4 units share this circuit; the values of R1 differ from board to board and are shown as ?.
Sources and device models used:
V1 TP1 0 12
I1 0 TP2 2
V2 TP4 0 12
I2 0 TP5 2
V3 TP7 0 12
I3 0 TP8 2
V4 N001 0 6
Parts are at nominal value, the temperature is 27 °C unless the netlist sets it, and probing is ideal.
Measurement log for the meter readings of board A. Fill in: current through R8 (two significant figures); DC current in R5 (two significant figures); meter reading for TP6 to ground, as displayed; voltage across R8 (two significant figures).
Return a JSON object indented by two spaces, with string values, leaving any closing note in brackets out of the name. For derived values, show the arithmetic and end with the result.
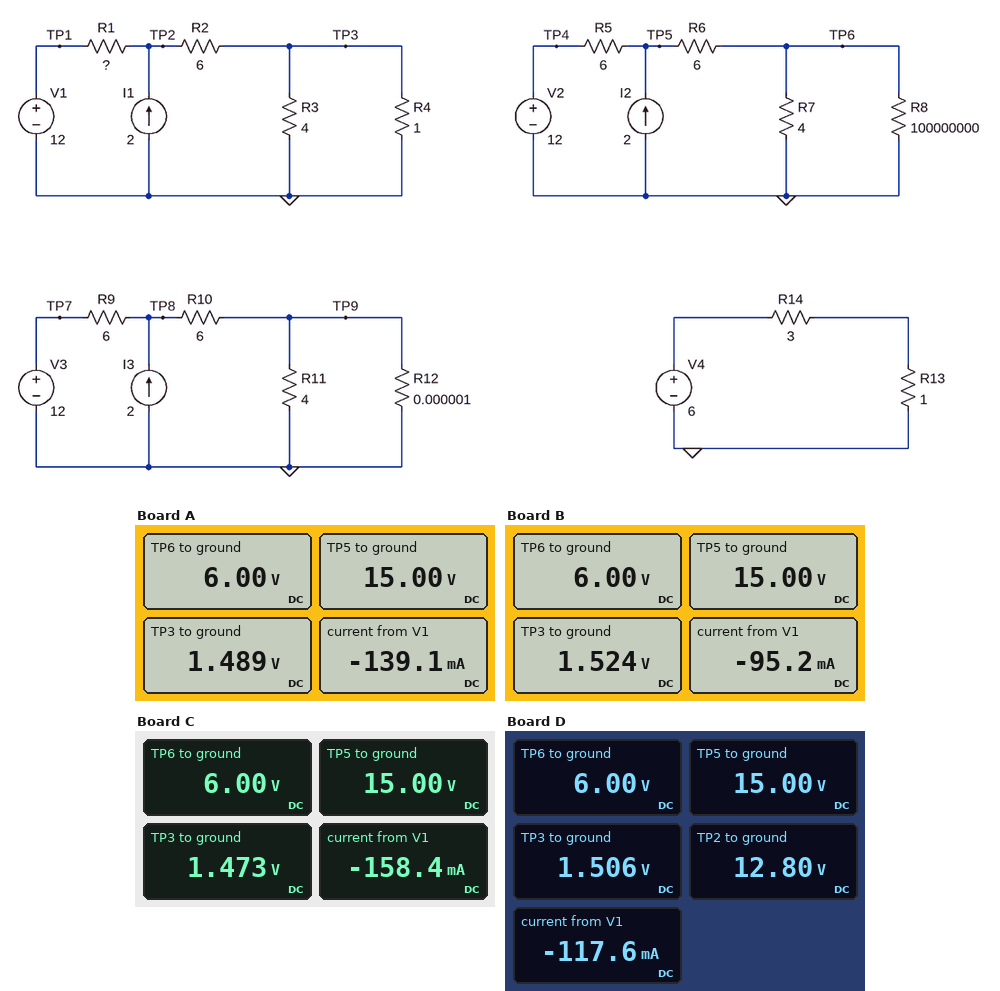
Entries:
{
  "current through R8": "(6 V) / 100 MΩ = 60 nA",
  "DC current in R5": "(15 V - 12 V) / 6 Ω = 500 mA",
  "meter reading for TP6 to ground, as displayed": "6.00 V",
  "voltage across R8": "6 V = 6.0 V"
}
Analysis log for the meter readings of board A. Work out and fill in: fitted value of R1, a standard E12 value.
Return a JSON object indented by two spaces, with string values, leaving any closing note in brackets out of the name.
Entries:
{
  "fitted value of R1, a standard E12 value": "4.7 Ω"
}
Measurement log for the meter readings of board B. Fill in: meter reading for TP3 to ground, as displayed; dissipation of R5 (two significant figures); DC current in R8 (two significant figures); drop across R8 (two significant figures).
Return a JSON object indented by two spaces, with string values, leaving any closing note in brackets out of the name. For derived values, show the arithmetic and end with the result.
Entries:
{
  "meter reading for TP3 to ground, as displayed": "1.524 V",
  "dissipation of R5": "(15 V - 12 V)^2 / 6 Ω = 1.5 W",
  "DC current in R8": "(6 V) / 100 MΩ = 60 nA",
  "drop across R8": "6 V = 6.0 V"
}
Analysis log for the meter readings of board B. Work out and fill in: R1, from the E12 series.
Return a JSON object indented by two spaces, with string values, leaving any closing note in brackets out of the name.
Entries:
{
  "R1, from the E12 series": "10 Ω"
}
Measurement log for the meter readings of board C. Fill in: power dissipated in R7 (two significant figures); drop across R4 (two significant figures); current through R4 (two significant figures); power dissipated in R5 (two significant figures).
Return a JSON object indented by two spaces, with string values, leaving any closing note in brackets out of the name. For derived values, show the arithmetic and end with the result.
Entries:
{
  "power dissipated in R7": "(6 V)^2 / 4 Ω = 9.0 W",
  "drop across R4": "1.473 V = 1.5 V",
  "current through R4": "(1.473 V) / 1 Ω = 1.5 A",
  "power dissipated in R5": "(15 V - 12 V)^2 / 6 Ω = 1.5 W"
}
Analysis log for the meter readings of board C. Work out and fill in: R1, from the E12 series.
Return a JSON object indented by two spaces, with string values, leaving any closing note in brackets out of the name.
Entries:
{
  "R1, from the E12 series": "3.3 Ω"
}
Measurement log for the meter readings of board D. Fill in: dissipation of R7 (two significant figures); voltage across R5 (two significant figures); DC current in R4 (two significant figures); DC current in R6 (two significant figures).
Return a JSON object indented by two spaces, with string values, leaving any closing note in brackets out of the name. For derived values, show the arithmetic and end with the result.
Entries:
{
  "dissipation of R7": "(6 V)^2 / 4 Ω = 9.0 W",
  "voltage across R5": "15 V - 12 V = 3.0 V",
  "DC current in R4": "(1.506 V) / 1 Ω = 1.5 A",
  "DC current in R6": "(15 V - 6 V) / 6 Ω = 1.5 A"
}
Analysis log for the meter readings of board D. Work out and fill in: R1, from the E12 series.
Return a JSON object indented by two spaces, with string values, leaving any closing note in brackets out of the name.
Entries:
{
  "R1, from the E12 series": "6.8 Ω"
}
